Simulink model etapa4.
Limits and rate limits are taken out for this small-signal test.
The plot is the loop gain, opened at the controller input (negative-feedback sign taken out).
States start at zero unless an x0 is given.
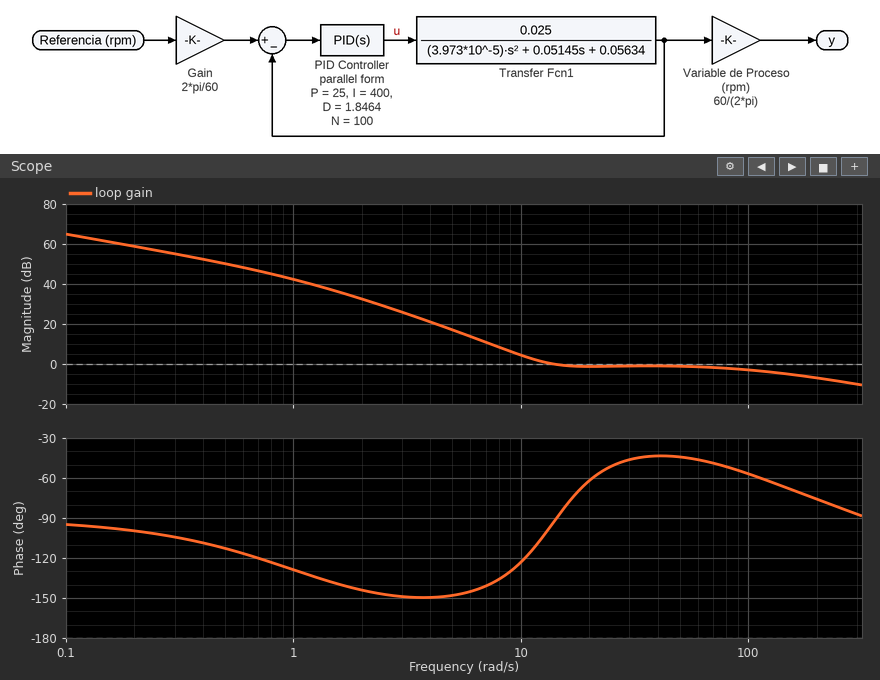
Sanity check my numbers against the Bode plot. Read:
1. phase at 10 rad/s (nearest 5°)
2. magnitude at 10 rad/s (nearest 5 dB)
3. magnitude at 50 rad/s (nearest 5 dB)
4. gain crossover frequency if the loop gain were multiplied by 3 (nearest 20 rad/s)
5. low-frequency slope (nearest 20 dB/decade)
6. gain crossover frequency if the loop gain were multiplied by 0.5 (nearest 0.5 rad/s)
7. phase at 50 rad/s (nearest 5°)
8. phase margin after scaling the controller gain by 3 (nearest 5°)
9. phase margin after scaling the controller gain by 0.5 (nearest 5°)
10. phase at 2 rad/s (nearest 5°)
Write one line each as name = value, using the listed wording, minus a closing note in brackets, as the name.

phase at 10 rad/s = -125°
magnitude at 10 rad/s = 5 dB
magnitude at 50 rad/s = 0 dB
gain crossover frequency if the loop gain were multiplied by 3 = 280 rad/s
low-frequency slope = -20 dB/decade
gain crossover frequency if the loop gain were multiplied by 0.5 = 9.0 rad/s
phase at 50 rad/s = -45°
phase margin after scaling the controller gain by 3 = 95°
phase margin after scaling the controller gain by 0.5 = 50°
phase at 2 rad/s = -145°
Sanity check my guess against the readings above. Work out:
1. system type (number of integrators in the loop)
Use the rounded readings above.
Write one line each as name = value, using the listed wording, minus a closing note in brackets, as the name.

system type = 1
